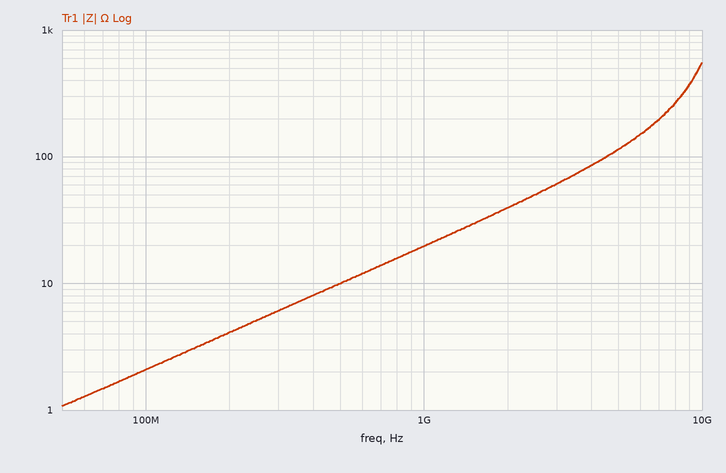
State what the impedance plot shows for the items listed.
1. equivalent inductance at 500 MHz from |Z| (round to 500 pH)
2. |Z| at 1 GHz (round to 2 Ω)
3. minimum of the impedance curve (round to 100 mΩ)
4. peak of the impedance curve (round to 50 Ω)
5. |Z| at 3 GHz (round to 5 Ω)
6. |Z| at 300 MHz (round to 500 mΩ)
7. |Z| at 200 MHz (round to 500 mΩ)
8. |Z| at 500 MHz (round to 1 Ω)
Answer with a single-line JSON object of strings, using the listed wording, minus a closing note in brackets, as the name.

{"equivalent inductance at 500 MHz from |Z|": "3.0 nH", "|Z| at 1 GHz": "20 Ω", "minimum of the impedance curve": "1.1 Ω", "peak of the impedance curve": "550 Ω", "|Z| at 3 GHz": "60 Ω", "|Z| at 300 MHz": "6.0 Ω", "|Z| at 200 MHz": "4.0 Ω", "|Z| at 500 MHz": "10 Ω"}
